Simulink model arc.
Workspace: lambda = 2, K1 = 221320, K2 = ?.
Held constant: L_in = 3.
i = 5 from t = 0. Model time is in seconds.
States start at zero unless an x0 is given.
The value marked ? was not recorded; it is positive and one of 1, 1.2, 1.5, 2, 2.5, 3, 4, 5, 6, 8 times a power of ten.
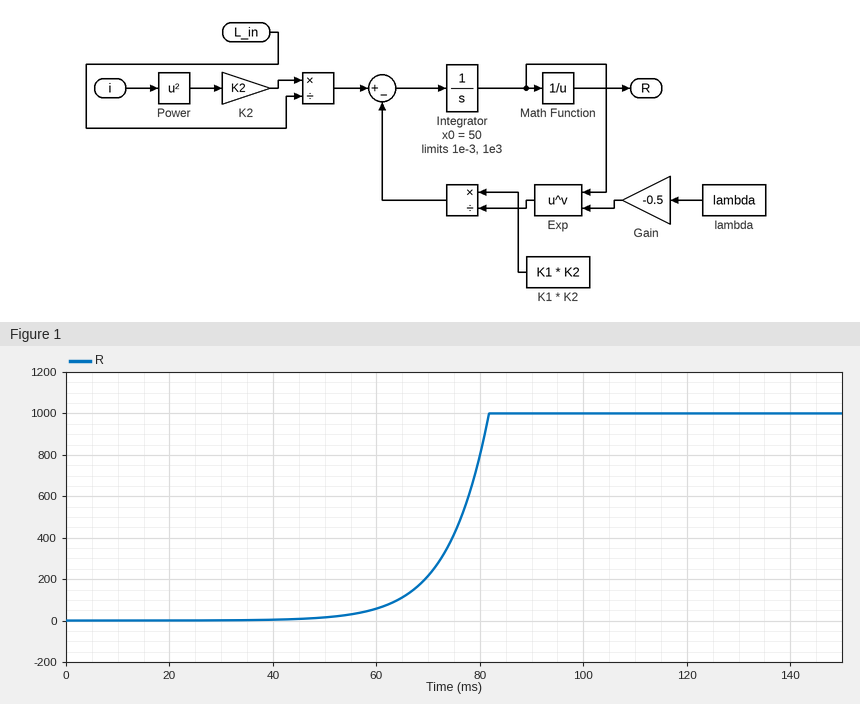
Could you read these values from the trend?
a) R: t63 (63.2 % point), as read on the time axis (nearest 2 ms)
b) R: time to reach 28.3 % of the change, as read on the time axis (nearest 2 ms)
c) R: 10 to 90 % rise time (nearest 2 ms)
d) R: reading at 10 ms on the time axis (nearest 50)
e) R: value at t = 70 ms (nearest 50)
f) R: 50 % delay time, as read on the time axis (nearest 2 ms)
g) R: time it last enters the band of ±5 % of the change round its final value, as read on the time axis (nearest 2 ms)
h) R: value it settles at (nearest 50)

78 ms
72 ms
16 ms
0
200
76 ms
82 ms
1000
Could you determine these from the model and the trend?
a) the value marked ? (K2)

0.0006
